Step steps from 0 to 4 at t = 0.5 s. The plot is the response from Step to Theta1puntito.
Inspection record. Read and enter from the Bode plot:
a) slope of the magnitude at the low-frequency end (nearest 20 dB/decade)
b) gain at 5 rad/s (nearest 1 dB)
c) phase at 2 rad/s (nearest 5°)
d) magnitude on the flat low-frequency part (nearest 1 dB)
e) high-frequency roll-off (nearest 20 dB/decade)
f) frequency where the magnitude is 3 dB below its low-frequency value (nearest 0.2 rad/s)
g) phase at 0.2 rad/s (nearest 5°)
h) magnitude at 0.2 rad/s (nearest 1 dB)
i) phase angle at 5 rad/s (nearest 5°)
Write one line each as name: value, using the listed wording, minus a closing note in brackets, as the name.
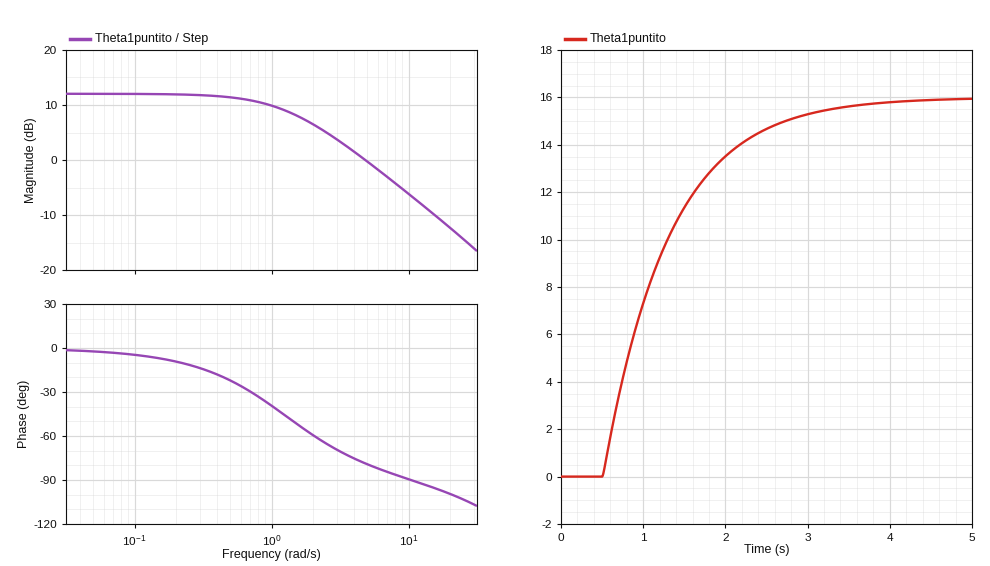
slope of the magnitude at the low-frequency end: 0 dB/decade
gain at 5 rad/s: 0 dB
phase at 2 rad/s: -60°
magnitude on the flat low-frequency part: 12 dB
high-frequency roll-off: -20 dB/decade
frequency where the magnitude is 3 dB below its low-frequency value: 1.2 rad/s
phase at 0.2 rad/s: -10°
magnitude at 0.2 rad/s: 12 dB
phase angle at 5 rad/s: -80°
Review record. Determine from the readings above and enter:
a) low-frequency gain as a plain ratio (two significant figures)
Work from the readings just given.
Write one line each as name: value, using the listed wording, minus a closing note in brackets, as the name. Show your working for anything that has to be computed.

low-frequency gain as a plain ratio: 10^(12 / 20) = 4.0
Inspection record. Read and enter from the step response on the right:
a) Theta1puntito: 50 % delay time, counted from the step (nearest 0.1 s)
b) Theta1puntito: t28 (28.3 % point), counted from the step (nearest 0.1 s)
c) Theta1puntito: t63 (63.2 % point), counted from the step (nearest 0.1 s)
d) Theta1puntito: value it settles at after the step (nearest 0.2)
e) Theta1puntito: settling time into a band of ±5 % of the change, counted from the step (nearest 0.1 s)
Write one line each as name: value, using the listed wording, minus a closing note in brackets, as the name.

Theta1puntito: 50 % delay time, counted from the step: 0.6 s
Theta1puntito: t28 (28.3 % point), counted from the step: 0.3 s
Theta1puntito: t63 (63.2 % point), counted from the step: 0.8 s
Theta1puntito: value it settles at after the step: 16.0
Theta1puntito: settling time into a band of ±5 % of the change, counted from the step: 2.4 s
